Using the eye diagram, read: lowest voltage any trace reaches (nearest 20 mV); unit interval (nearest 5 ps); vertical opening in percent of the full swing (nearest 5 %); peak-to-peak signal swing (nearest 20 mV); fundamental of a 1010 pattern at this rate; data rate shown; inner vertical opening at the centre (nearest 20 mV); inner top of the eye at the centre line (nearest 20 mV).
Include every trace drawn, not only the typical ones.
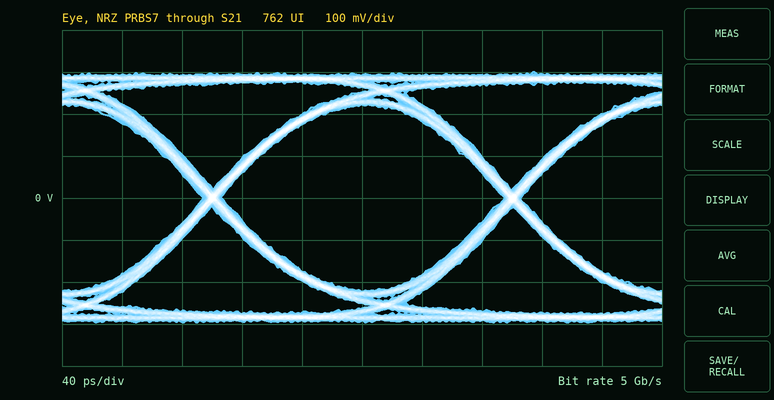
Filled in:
-300 mV
200 ps
75 %
600 mV
2.5 GHz
5 Gb/s
440 mV
220 mV
